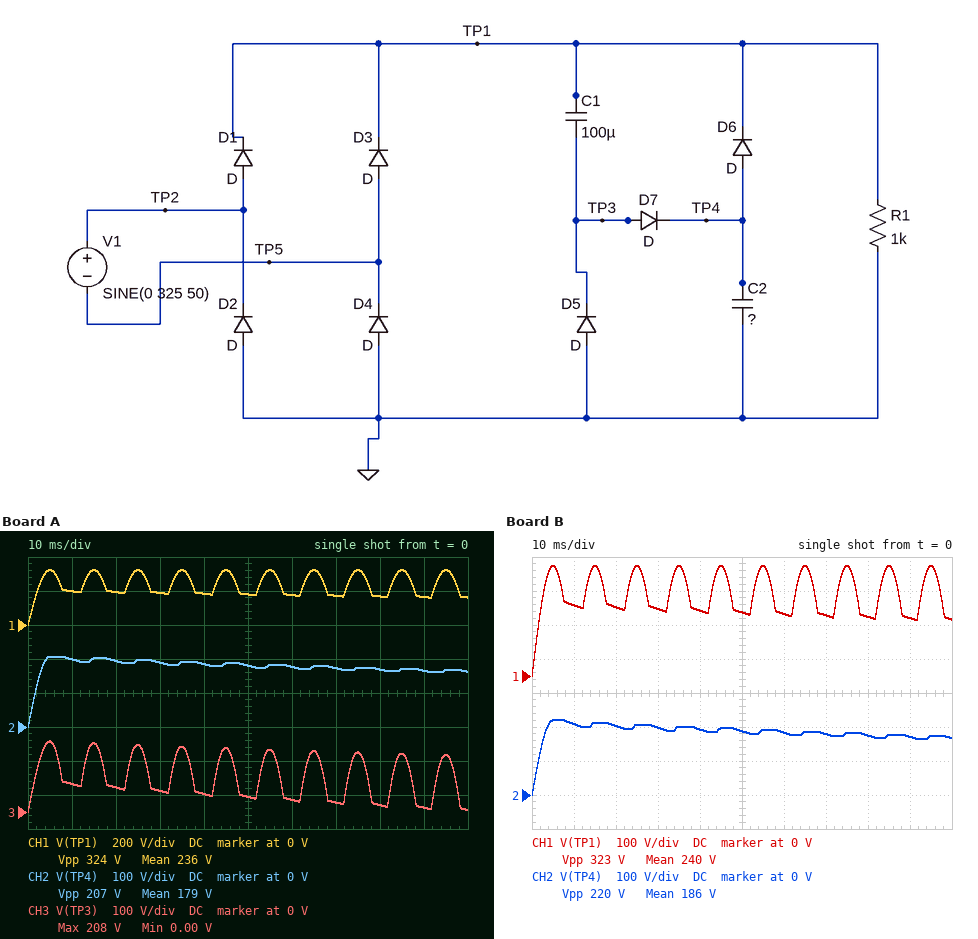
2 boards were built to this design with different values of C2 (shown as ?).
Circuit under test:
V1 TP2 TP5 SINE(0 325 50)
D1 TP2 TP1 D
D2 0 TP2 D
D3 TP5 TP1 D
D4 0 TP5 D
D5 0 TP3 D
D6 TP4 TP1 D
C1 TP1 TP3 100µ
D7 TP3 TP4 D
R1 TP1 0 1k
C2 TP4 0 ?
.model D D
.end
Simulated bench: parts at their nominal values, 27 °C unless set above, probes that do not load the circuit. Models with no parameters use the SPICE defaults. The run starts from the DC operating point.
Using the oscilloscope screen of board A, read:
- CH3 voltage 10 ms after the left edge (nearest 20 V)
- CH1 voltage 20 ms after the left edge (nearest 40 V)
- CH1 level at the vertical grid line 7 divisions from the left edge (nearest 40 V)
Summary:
80 V
200 V
160 V
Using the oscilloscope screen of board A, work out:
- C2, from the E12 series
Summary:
56 µF
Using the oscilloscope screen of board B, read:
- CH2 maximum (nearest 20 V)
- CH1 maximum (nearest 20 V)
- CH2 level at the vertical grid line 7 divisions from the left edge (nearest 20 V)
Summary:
220 V
320 V
180 V
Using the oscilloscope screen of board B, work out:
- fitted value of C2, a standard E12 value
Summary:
47 µF
